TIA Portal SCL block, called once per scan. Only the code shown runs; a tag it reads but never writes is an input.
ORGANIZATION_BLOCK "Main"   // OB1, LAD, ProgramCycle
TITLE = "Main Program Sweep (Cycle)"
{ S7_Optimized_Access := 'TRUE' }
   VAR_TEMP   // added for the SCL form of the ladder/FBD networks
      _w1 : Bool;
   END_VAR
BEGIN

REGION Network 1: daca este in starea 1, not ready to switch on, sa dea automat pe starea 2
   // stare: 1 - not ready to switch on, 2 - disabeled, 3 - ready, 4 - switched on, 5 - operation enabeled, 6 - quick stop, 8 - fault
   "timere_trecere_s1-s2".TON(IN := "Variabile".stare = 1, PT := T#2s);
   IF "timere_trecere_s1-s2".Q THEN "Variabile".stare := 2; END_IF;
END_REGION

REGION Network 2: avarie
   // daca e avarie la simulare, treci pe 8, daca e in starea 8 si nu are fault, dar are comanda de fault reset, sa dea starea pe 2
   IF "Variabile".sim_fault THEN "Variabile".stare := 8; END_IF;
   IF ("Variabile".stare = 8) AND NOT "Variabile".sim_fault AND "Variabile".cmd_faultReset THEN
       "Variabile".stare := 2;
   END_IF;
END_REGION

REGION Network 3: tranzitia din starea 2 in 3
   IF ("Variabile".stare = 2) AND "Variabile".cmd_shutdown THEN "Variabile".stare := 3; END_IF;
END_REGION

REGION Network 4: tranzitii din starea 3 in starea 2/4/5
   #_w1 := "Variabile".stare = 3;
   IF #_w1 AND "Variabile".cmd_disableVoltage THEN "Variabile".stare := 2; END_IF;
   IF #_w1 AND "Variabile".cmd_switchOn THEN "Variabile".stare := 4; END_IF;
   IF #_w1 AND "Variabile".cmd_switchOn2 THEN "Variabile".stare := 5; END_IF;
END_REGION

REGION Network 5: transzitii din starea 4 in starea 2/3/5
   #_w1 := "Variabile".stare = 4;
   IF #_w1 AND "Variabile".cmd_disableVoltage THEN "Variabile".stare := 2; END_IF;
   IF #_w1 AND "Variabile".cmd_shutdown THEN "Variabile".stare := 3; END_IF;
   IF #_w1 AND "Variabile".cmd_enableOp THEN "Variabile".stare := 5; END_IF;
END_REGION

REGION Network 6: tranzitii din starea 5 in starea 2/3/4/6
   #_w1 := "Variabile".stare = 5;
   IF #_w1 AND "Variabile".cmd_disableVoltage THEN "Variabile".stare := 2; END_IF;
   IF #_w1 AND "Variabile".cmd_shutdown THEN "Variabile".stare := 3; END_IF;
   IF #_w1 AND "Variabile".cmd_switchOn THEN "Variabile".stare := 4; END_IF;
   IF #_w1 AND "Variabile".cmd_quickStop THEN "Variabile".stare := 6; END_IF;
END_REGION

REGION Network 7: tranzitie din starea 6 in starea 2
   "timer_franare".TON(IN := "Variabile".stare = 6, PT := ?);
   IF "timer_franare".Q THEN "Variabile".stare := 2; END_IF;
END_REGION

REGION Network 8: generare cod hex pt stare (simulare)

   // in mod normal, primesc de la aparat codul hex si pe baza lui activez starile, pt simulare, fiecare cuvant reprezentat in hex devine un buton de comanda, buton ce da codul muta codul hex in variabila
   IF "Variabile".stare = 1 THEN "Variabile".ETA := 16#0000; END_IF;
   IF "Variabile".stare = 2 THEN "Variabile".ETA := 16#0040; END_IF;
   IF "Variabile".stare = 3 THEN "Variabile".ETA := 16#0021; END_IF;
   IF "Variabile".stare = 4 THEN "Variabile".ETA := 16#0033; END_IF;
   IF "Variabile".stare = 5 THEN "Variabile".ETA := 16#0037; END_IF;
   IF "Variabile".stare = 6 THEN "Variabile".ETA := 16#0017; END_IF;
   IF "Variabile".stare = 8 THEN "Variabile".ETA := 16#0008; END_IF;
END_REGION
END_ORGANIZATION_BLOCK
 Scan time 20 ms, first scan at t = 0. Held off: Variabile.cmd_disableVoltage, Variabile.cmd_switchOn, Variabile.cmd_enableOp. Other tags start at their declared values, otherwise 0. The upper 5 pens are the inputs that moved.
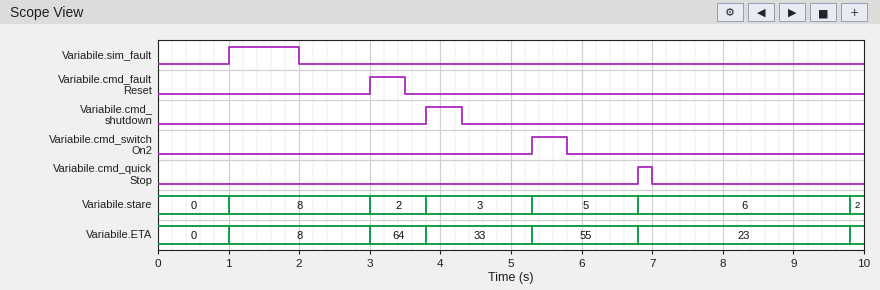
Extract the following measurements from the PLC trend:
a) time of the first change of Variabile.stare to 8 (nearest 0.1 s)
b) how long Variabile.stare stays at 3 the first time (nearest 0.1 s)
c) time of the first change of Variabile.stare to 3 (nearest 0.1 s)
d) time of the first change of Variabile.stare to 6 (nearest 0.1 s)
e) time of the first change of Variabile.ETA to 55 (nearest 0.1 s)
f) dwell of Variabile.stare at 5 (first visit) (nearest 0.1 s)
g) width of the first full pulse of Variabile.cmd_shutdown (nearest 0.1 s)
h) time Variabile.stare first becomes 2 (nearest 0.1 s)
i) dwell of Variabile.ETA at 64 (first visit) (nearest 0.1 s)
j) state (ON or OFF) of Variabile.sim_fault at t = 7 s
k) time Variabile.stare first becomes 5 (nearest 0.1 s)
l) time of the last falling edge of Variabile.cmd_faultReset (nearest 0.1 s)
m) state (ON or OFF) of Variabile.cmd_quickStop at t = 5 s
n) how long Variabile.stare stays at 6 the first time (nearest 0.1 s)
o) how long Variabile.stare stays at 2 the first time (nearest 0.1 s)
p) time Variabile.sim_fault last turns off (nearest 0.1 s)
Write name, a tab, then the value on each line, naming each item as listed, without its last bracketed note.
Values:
time of the first change of Variabile.stare to 8	1.0 s
how long Variabile.stare stays at 3 the first time	1.5 s
time of the first change of Variabile.stare to 3	3.8 s
time of the first change of Variabile.stare to 6	6.8 s
time of the first change of Variabile.ETA to 55	5.3 s
dwell of Variabile.stare at 5 (first visit)	1.5 s
width of the first full pulse of Variabile.cmd_shutdown	0.5 s
time Variabile.stare first becomes 2	3.0 s
dwell of Variabile.ETA at 64 (first visit)	0.8 s
state (ON or OFF) of Variabile.sim_fault at t = 7 s	OFF
time Variabile.stare first becomes 5	5.3 s
time of the last falling edge of Variabile.cmd_faultReset	3.5 s
state (ON or OFF) of Variabile.cmd_quickStop at t = 5 s	OFF
how long Variabile.stare stays at 6 the first time	3.0 s
how long Variabile.stare stays at 2 the first time	0.8 s
time Variabile.sim_fault last turns off	2.0 s
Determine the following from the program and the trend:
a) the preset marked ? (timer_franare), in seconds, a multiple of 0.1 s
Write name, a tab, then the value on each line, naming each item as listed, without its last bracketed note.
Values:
the preset marked ? (timer_franare), in seconds, a multiple of 0.1 s	3.0 s
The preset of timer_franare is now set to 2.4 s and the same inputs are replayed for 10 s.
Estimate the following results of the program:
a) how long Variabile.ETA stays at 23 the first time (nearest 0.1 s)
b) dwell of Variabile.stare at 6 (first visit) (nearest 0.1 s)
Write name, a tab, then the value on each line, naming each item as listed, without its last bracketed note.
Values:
how long Variabile.ETA stays at 23 the first time	2.4 s
dwell of Variabile.stare at 6 (first visit)	2.4 s
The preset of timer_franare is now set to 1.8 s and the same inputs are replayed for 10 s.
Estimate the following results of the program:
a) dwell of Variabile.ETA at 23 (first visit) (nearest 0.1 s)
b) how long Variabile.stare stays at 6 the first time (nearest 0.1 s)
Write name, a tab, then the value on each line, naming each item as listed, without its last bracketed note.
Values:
dwell of Variabile.ETA at 23 (first visit)	1.8 s
how long Variabile.stare stays at 6 the first time	1.8 s
